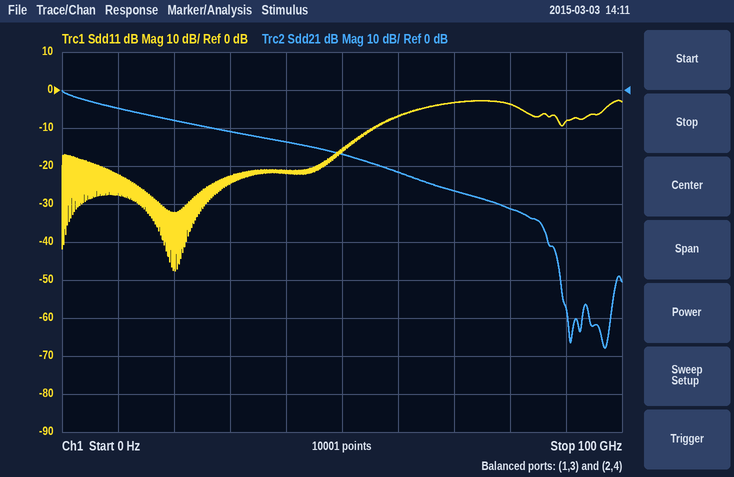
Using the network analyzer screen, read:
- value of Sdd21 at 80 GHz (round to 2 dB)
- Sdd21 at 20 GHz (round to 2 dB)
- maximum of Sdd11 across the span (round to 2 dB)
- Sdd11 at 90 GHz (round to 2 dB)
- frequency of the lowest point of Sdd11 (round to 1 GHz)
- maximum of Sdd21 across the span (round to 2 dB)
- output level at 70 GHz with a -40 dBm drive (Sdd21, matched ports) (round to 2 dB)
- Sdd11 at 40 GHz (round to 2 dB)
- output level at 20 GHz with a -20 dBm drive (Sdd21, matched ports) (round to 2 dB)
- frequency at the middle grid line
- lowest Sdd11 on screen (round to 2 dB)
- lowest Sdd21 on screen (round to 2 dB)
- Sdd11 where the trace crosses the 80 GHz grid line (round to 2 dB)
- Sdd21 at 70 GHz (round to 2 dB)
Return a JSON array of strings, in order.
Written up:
["-32 dB", "-8 dB", "-2 dB", "-8 dB", "20 GHz", "0 dB", "-66 dBm", "-22 dB", "-28 dBm", "50 GHz", "-48 dB", "-68 dB", "-4 dB", "-26 dB"]
